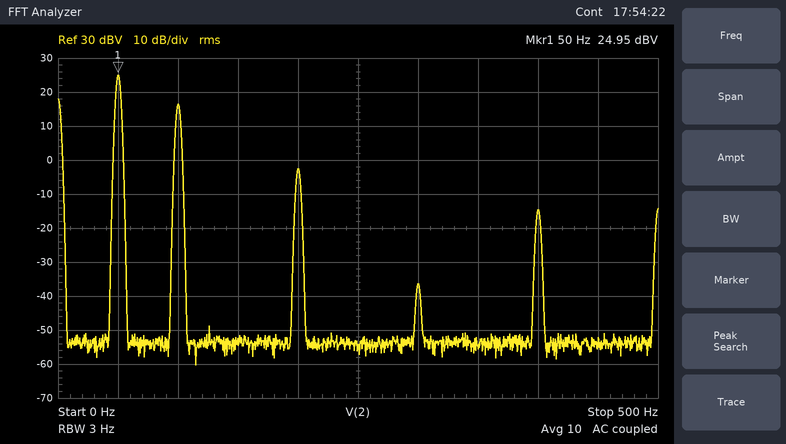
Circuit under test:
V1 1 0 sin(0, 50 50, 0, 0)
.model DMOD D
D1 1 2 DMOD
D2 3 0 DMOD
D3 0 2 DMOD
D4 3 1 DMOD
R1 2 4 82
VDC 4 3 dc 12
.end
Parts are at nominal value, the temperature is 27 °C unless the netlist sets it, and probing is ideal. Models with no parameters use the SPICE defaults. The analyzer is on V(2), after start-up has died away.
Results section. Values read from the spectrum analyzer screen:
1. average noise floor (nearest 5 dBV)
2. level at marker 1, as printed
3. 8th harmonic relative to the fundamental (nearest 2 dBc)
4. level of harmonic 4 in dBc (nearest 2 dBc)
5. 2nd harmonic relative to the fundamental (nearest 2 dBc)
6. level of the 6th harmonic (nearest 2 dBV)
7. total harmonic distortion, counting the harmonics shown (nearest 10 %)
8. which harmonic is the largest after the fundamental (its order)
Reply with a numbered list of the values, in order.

1. -55 dBV
2. 24.95 dBV
3. -40 dBc
4. -28 dBc
5. -8 dBc
6. -36 dBV
7. 40 %
8. 2
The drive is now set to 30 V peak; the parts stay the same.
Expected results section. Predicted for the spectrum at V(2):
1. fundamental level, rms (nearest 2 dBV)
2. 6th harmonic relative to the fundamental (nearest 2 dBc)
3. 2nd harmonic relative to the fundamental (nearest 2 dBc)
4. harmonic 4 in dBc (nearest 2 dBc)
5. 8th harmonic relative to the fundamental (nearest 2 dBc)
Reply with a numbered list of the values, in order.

1. 20 dBV
2. -30 dBc
3. -10 dBc
4. -38 dBc
5. -36 dBc
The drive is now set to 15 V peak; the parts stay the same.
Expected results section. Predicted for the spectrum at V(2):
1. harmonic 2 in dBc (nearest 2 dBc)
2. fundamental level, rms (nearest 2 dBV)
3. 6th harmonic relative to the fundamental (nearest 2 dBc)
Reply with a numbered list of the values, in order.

1. -28 dBc
2. 14 dBV
3. -36 dBc
